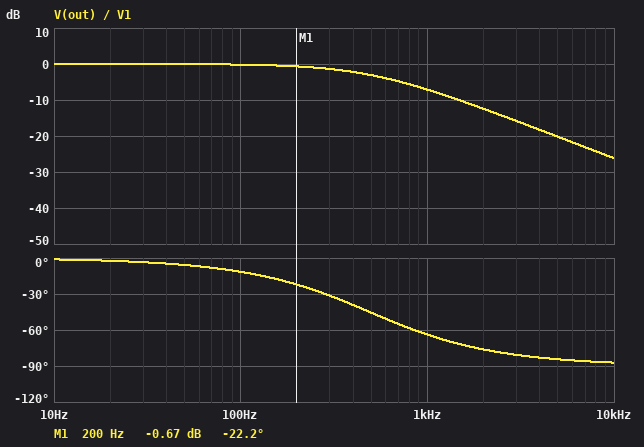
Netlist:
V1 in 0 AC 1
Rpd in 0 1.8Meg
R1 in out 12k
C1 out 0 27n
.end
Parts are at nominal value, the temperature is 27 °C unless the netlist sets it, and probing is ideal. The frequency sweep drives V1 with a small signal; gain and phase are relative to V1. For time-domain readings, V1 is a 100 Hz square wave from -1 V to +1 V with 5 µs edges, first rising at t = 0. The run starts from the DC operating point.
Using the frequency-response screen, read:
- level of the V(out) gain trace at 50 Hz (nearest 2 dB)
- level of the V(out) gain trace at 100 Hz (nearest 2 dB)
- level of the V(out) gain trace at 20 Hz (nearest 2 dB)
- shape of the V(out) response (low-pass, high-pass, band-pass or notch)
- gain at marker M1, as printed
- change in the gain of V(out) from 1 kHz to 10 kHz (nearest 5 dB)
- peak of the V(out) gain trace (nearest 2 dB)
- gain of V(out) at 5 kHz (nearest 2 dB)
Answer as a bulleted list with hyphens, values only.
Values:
- 0 dB
- 0 dB
- 0 dB
- low-pass
- -0.67 dB
- -20 dB
- 0 dB
- -20 dB
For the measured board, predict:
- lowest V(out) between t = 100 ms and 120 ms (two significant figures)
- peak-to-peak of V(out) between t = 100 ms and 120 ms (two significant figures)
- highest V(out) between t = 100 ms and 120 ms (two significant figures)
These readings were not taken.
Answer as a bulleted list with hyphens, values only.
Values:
- -1.0 V
- 2.0 V
- 1.0 V
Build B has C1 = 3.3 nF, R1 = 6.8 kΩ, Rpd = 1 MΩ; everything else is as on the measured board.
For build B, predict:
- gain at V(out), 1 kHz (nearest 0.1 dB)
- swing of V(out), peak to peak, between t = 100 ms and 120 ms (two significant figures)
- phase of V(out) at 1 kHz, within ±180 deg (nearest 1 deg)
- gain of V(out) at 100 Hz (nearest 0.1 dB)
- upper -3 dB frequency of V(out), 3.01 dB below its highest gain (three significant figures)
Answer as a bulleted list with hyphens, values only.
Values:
- -0.1 dB
- 2.0 V
- -8 deg
- 0 dB
- 7.09 kHz
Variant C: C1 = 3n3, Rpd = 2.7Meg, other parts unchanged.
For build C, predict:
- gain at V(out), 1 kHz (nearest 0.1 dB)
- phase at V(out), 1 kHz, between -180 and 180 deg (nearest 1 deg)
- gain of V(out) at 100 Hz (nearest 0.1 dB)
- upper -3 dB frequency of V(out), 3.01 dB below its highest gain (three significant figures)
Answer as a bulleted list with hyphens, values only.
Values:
- -0.3 dB
- -14 deg
- 0 dB
- 4.02 kHz
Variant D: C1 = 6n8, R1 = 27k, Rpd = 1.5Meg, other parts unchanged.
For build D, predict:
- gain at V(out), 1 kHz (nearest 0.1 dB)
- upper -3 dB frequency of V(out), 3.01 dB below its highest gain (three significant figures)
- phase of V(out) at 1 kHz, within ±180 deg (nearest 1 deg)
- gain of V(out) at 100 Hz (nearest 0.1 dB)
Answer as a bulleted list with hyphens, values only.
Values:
- -3.7 dB
- 867 Hz
- -49 deg
- -0.1 dB
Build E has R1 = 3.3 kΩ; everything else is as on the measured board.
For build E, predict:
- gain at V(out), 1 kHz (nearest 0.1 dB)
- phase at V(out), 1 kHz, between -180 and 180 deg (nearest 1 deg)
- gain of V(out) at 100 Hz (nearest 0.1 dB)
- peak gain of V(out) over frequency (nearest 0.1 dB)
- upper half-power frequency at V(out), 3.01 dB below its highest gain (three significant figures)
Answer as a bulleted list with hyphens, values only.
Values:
- -1.2 dB
- -29 deg
- 0 dB
- 0 dB
- 1.79 kHz
